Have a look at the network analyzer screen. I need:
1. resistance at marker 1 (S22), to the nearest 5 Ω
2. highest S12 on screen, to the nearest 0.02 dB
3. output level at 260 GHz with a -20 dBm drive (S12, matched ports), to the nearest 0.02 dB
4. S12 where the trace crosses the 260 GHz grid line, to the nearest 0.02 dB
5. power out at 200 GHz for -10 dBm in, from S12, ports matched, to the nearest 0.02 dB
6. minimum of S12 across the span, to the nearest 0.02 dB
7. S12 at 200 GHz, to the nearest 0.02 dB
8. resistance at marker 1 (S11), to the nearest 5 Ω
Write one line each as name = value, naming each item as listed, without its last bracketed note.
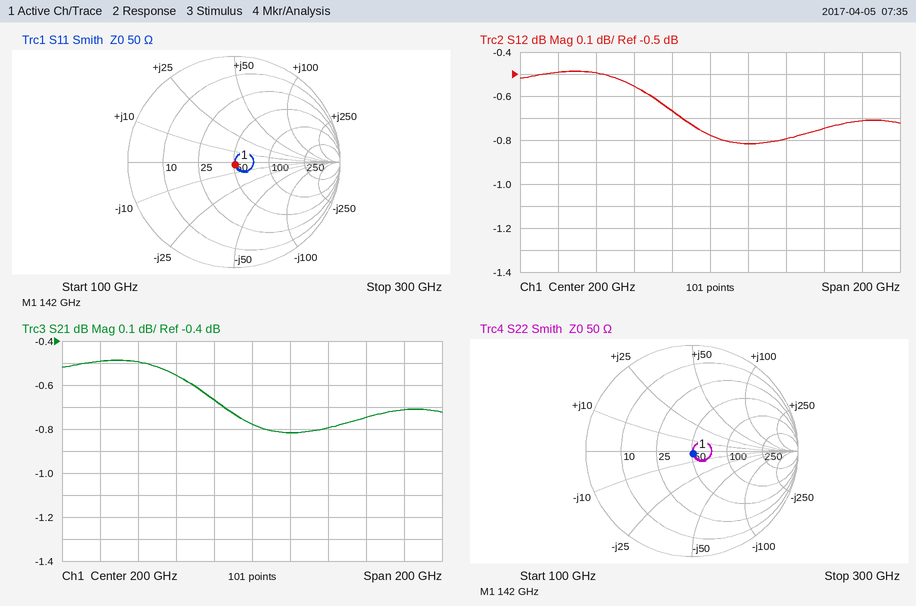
resistance at marker 1 (S22), to the nearest 5 Ω = 50 Ω
highest S12 on screen, to the nearest 0.02 dB = -0.48 dB
output level at 260 GHz with a -20 dBm drive (S12, matched ports), to the nearest 0.02 dB = -20.74 dBm
S12 where the trace crosses the 260 GHz grid line, to the nearest 0.02 dB = -0.74 dB
power out at 200 GHz for -10 dBm in, from S12, ports matched, to the nearest 0.02 dB = -10.78 dBm
minimum of S12 across the span, to the nearest 0.02 dB = -0.82 dB
S12 at 200 GHz, to the nearest 0.02 dB = -0.78 dB
resistance at marker 1 (S11), to the nearest 5 Ω = 50 Ω
